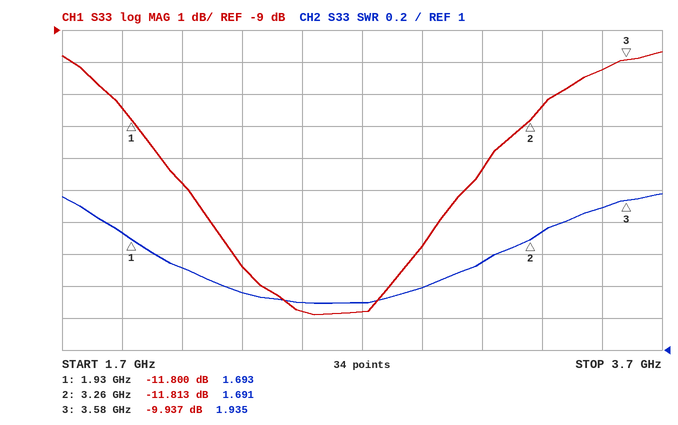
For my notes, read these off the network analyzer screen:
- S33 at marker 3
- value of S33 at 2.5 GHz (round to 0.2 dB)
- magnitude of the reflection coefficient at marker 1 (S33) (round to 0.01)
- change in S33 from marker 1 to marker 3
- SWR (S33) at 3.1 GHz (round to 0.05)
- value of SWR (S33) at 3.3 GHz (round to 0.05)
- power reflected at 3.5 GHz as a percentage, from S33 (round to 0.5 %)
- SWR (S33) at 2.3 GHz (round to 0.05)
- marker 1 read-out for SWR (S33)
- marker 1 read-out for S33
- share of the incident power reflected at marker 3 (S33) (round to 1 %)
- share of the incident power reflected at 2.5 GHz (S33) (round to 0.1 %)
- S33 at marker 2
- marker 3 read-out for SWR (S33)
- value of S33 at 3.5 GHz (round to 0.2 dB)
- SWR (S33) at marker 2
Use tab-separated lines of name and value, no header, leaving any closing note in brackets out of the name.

S33 at marker 3	-9.937 dB
value of S33 at 2.5 GHz	-17.8 dB
magnitude of the reflection coefficient at marker 1 (S33)	0.26
change in S33 from marker 1 to marker 3	1.863 dB
SWR (S33) at 3.1 GHz	1.55
value of SWR (S33) at 3.3 GHz	1.75
power reflected at 3.5 GHz as a percentage, from S33	9.5 %
SWR (S33) at 2.3 GHz	1.35
marker 1 read-out for SWR	1.693
marker 1 read-out for S33	-11.800 dB
share of the incident power reflected at marker 3 (S33)	10 %
share of the incident power reflected at 2.5 GHz (S33)	1.7 %
S33 at marker 2	-11.813 dB
marker 3 read-out for SWR	1.935
value of S33 at 3.5 GHz	-10.2 dB
SWR (S33) at marker 2	1.691
